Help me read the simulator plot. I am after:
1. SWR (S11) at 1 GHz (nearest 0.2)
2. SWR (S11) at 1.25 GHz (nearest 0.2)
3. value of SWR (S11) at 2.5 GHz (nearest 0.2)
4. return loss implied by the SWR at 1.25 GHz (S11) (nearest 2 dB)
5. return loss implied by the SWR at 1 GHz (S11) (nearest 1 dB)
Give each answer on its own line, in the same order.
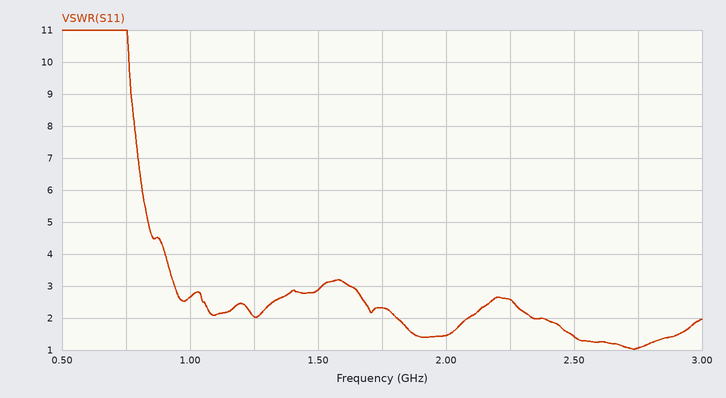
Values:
2.6
2.0
1.4
10 dB
7 dB
